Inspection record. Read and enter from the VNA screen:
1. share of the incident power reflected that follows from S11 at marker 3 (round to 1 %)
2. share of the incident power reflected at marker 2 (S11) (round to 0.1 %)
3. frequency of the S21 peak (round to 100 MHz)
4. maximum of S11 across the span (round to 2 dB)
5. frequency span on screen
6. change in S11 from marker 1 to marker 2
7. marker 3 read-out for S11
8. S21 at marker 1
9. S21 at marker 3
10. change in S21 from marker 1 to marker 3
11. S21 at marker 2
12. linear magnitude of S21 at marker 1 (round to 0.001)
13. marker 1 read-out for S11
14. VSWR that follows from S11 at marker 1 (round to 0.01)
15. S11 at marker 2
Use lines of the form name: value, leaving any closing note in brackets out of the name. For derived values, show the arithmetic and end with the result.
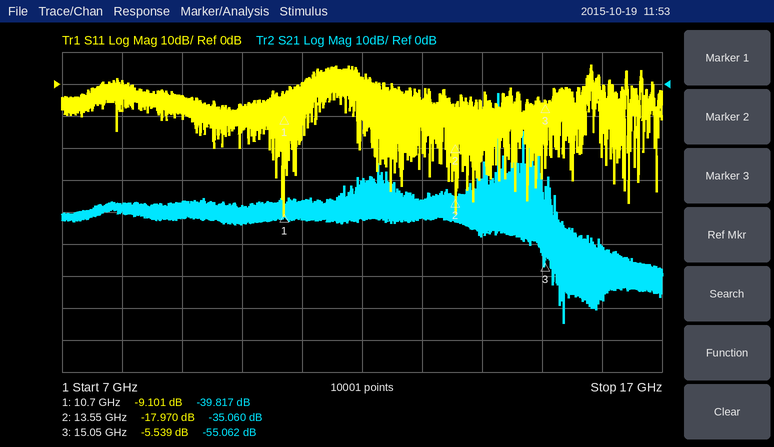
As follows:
share of the incident power reflected that follows from S11 at marker 3: 10^(-5.539/10) ≈ 28 %
share of the incident power reflected at marker 2 (S11): 10^(-17.97/10) ≈ 1.6 %
frequency of the S21 peak: 14.3 GHz
maximum of S11 across the span: 6 dB
frequency span on screen: 10 GHz
change in S11 from marker 1 to marker 2: -17.97 − (-9.101) = -8.869 dB
marker 3 read-out for S11: -5.539 dB
S21 at marker 1: -39.817 dB
S21 at marker 3: -55.062 dB
change in S21 from marker 1 to marker 3: -55.062 − (-39.817) = -15.245 dB
S21 at marker 2: -35.060 dB
linear magnitude of S21 at marker 1: 10^(-39.817/20) ≈ 0.010
marker 1 read-out for S11: -9.101 dB
VSWR that follows from S11 at marker 1: (1 + 0.3507)/(1 − 0.3507) ≈ 2.08
S11 at marker 2: -17.970 dB
